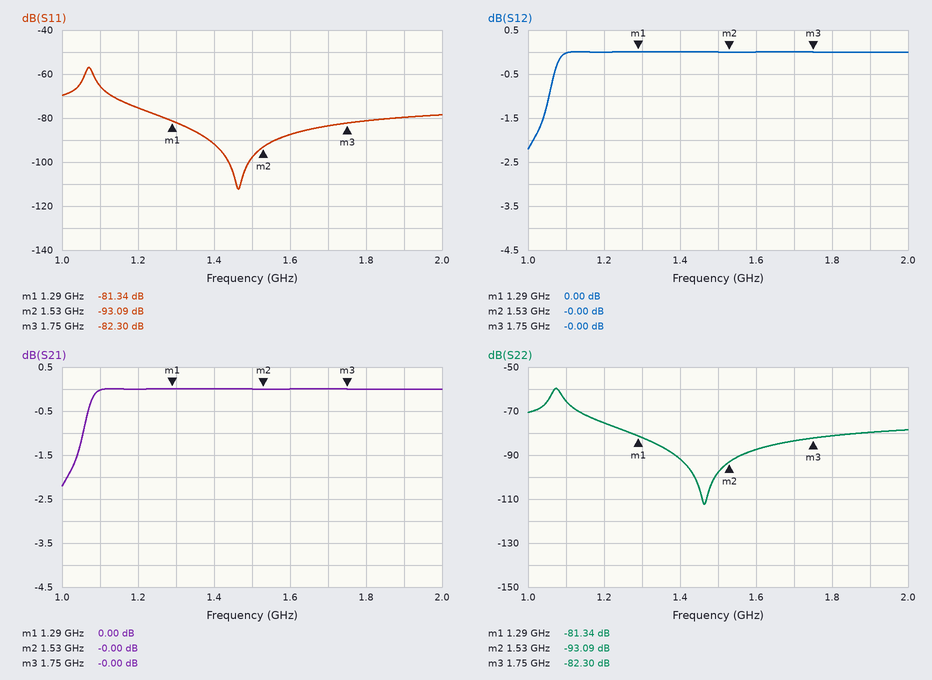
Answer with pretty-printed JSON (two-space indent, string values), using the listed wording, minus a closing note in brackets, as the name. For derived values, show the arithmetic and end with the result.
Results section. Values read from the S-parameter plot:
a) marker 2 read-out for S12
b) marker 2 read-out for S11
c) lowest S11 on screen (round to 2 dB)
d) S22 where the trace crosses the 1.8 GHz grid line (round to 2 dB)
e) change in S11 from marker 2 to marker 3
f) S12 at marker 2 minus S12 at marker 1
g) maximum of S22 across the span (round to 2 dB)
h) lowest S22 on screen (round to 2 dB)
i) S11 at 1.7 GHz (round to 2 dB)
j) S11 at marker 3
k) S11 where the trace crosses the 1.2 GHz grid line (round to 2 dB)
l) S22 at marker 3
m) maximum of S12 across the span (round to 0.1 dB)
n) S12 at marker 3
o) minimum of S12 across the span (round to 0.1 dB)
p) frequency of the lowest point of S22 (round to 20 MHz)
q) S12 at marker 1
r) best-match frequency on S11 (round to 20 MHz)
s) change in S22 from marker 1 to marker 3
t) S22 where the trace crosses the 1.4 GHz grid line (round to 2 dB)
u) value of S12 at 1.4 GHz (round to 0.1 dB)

{
  "marker 2 read-out for S12": "-0.00 dB",
  "marker 2 read-out for S11": "-93.09 dB",
  "lowest S11 on screen": "-112 dB",
  "S22 where the trace crosses the 1.8 GHz grid line": "-82 dB",
  "change in S11 from marker 2 to marker 3": "-82.3 − (-93.09) = 10.79 dB",
  "S12 at marker 2 minus S12 at marker 1": "-0 − (0) = 0.00 dB",
  "maximum of S22 across the span": "-60 dB",
  "lowest S22 on screen": "-112 dB",
  "S11 at 1.7 GHz": "-84 dB",
  "S11 at marker 3": "-82.30 dB",
  "S11 where the trace crosses the 1.2 GHz grid line": "-76 dB",
  "S22 at marker 3": "-82.30 dB",
  "maximum of S12 across the span": "0.0 dB",
  "S12 at marker 3": "-0.00 dB",
  "minimum of S12 across the span": "-2.2 dB",
  "frequency of the lowest point of S22": "1.46 GHz",
  "S12 at marker 1": "0.00 dB",
  "best-match frequency on S11": "1.46 GHz",
  "change in S22 from marker 1 to marker 3": "-82.3 − (-81.34) = -0.96 dB",
  "S22 where the trace crosses the 1.4 GHz grid line": "-92 dB",
  "value of S12 at 1.4 GHz": "0.0 dB"
}
